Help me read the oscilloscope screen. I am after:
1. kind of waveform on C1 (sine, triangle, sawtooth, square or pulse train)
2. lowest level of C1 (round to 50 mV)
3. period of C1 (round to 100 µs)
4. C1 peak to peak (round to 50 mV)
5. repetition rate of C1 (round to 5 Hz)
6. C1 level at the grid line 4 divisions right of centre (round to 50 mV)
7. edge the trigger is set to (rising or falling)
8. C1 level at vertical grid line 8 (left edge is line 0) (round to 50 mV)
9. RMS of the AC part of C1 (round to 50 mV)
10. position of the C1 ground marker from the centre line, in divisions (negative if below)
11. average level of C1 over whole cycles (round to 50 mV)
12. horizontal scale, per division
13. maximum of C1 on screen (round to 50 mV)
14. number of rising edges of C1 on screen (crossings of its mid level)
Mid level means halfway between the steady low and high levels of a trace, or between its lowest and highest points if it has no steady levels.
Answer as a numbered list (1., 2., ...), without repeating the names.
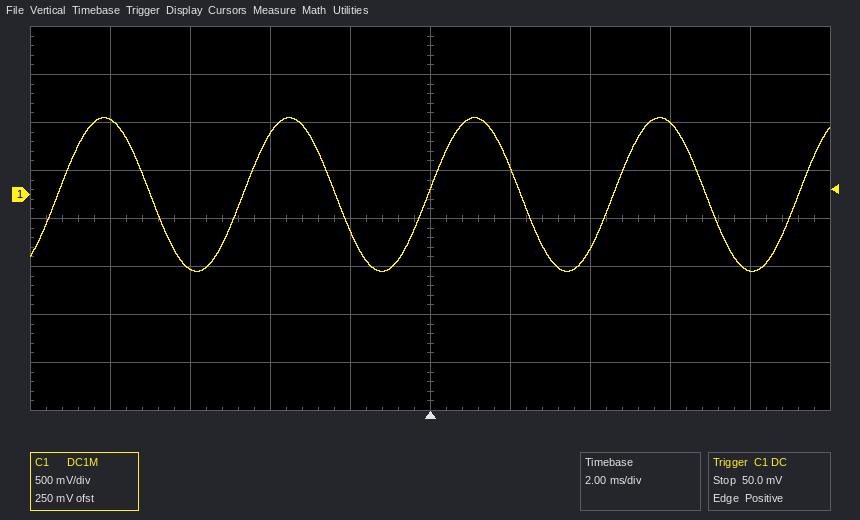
1. sine
2. -800 mV
3. 4.6 ms
4. 1.60 V
5. 215 Hz
6. -800 mV
7. rising
8. 750 mV
9. 550 mV
10. +0.5 div
11. 0 mV
12. 2 ms
13. 800 mV
14. 5
